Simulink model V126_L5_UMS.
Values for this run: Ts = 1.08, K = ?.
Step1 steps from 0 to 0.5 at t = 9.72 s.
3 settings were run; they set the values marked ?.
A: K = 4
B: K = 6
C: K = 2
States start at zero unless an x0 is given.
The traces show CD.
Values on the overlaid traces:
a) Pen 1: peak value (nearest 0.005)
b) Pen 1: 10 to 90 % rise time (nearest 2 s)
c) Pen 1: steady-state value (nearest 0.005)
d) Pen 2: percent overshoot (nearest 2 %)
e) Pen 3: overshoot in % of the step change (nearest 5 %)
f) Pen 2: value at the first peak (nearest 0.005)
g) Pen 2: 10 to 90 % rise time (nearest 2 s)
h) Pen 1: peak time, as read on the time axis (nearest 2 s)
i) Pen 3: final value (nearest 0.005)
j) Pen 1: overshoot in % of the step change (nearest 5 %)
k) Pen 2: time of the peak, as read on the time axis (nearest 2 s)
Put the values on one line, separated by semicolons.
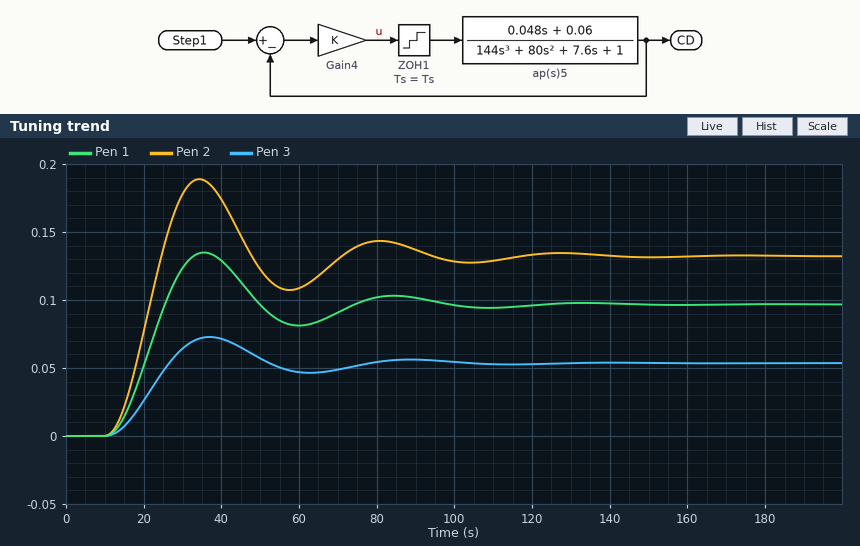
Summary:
0.135; 10 s; 0.095; 42 %; 35 %; 0.190; 10 s; 36 s; 0.055; 40 %; 34 s
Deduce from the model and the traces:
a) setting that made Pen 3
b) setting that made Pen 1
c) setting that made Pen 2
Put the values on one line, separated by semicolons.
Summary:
C; A; B
